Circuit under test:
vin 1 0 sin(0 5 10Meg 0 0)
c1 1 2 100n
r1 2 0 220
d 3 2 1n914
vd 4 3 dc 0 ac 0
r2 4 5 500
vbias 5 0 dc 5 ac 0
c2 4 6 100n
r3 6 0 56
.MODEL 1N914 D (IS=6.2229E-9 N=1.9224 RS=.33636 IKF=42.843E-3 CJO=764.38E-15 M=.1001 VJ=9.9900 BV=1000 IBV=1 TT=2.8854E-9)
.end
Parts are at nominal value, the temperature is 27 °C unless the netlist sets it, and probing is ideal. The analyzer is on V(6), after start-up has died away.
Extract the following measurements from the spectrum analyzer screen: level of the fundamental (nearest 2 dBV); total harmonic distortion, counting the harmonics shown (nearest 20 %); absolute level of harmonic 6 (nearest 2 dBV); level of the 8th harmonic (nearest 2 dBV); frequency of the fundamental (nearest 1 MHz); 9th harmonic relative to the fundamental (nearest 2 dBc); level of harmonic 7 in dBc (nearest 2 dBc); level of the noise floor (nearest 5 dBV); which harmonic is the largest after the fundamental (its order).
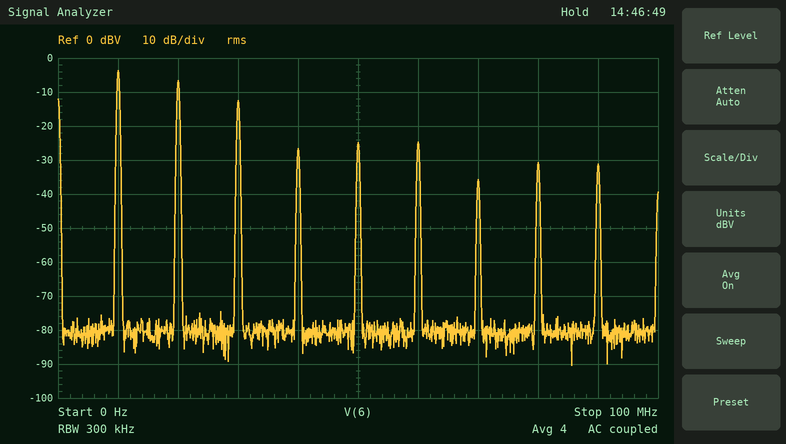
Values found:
-4 dBV
80 %
-24 dBV
-30 dBV
10 MHz
-28 dBc
-32 dBc
-80 dBV
2
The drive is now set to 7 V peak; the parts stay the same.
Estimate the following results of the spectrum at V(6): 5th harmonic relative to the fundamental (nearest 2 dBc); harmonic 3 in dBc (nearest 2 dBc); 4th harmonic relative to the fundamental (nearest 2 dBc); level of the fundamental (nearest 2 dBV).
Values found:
-24 dBc
-8 dBc
-18 dBc
-2 dBV
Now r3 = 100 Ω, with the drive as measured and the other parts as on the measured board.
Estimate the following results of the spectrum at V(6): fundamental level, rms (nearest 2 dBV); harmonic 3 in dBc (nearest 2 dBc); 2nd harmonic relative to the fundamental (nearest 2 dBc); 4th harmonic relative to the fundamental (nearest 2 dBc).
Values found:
0 dBV
-14 dBc
-4 dBc
-26 dBc
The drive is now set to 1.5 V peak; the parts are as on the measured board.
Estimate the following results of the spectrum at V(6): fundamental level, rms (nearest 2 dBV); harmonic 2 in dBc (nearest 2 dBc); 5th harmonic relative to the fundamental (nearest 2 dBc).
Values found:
-8 dBV
-6 dBc
-30 dBc
